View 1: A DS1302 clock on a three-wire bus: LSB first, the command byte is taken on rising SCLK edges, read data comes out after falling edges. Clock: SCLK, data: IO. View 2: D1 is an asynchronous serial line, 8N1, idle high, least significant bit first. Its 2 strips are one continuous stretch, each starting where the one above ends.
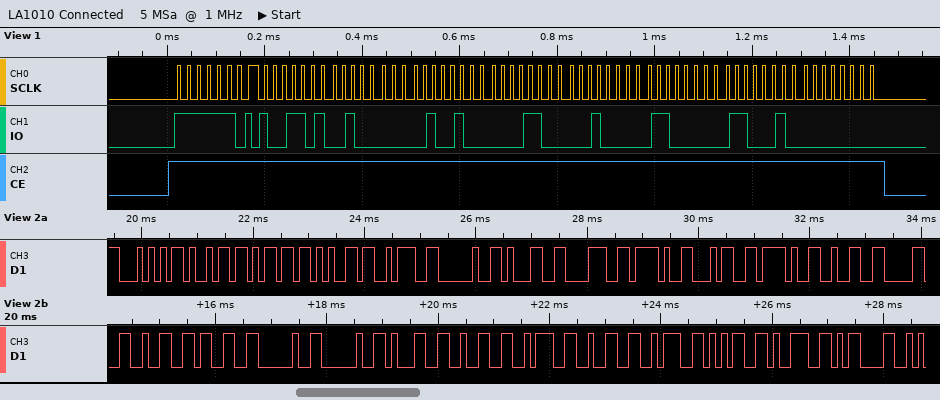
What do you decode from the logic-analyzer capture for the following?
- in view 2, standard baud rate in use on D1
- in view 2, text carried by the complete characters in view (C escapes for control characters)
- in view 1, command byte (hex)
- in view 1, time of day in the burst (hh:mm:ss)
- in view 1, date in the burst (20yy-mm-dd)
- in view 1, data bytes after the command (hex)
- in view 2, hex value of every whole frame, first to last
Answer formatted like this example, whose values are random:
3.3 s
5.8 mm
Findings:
9600 baud
"Time: 18/4/2023  12:2:59\r"
0xBF
12:02:59
2023-04-18
59 02 12 18 04 03 23 00
54 69 6D 65 3A 20 31 38 2F 34 2F 32 30 32 33 20 20 31 32 3A 32 3A 35 39 0D
